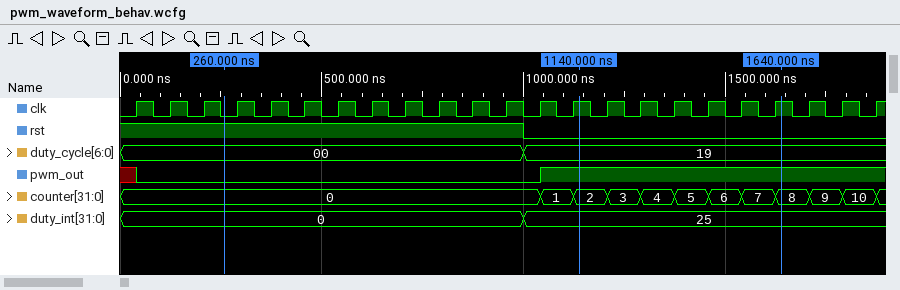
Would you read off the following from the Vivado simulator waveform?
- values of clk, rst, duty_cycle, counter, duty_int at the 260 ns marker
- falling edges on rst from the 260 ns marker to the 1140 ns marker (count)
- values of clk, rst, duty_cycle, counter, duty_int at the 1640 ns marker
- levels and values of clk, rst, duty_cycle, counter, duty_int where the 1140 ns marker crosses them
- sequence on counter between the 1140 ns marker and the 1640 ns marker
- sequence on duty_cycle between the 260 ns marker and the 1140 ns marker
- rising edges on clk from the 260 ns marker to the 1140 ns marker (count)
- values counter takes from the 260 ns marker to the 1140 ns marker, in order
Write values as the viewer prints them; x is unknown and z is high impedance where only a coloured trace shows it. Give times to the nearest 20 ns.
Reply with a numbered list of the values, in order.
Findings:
1. clk=0, rst=1, duty_cycle=00, counter=0, duty_int=0
2. 1
3. clk=1, rst=0, duty_cycle=19, counter=8, duty_int=25
4. clk=1, rst=0, duty_cycle=19, counter=2, duty_int=25
5. 2, 3, 4, 5, 6, 7, 8
6. 00, 19
7. 11
8. 0, 1, 2
